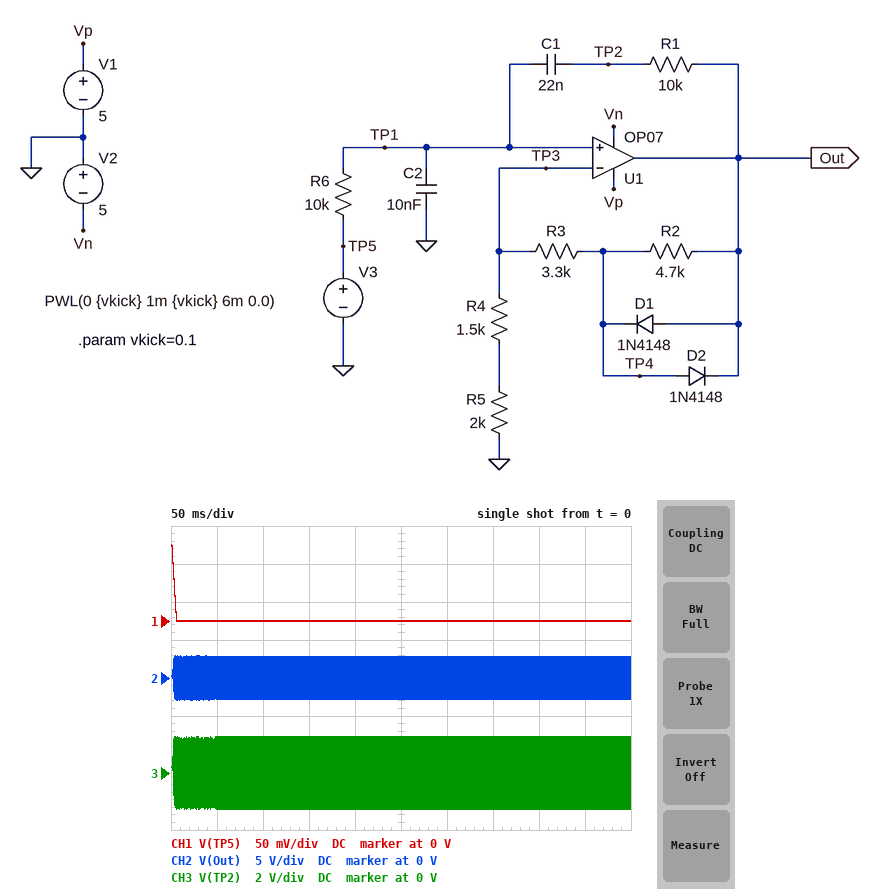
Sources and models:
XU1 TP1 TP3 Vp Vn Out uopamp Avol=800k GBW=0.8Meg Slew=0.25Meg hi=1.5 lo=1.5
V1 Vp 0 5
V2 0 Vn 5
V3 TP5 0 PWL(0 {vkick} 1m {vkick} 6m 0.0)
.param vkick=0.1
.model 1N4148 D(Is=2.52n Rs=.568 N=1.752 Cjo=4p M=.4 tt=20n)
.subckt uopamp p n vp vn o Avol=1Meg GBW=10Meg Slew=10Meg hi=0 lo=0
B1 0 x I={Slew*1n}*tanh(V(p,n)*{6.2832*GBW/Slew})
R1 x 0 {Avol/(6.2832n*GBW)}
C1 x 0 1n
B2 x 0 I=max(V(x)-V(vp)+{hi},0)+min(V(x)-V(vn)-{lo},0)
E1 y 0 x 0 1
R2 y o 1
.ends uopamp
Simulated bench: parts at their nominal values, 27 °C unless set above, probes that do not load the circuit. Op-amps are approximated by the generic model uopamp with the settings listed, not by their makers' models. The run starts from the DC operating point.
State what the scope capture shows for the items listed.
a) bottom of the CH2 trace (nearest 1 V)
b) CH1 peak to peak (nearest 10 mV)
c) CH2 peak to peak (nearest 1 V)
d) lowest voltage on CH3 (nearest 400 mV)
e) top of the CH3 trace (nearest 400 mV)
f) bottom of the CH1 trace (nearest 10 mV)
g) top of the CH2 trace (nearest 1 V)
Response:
-3 V
100 mV
6 V
-2.0 V
2.0 V
0 V
3 V
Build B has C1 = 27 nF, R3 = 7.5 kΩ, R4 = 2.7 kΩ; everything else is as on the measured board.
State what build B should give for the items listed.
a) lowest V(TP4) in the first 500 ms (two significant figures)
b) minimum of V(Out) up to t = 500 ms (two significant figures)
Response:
-3.0 V
-3.5 V
